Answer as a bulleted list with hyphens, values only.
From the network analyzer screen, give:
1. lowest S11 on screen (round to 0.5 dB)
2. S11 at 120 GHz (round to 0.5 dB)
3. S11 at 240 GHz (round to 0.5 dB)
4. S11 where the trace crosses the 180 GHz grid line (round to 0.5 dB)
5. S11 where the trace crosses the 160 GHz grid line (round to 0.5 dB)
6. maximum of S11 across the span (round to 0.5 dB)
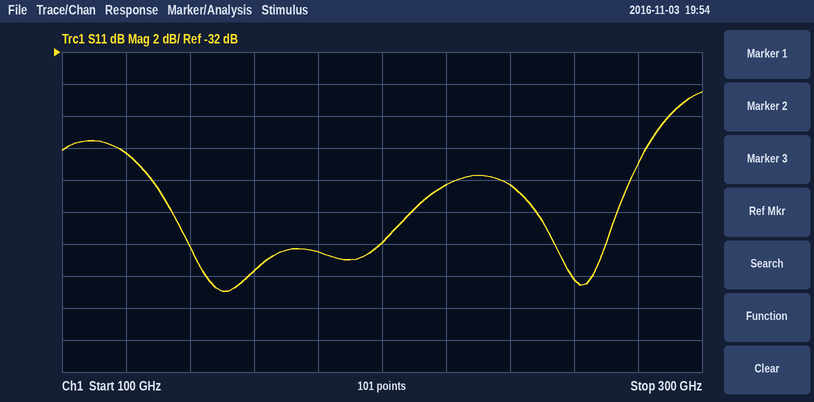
- -47.0 dB
- -38.5 dB
- -40.5 dB
- -44.5 dB
- -45.5 dB
- -34.5 dB
